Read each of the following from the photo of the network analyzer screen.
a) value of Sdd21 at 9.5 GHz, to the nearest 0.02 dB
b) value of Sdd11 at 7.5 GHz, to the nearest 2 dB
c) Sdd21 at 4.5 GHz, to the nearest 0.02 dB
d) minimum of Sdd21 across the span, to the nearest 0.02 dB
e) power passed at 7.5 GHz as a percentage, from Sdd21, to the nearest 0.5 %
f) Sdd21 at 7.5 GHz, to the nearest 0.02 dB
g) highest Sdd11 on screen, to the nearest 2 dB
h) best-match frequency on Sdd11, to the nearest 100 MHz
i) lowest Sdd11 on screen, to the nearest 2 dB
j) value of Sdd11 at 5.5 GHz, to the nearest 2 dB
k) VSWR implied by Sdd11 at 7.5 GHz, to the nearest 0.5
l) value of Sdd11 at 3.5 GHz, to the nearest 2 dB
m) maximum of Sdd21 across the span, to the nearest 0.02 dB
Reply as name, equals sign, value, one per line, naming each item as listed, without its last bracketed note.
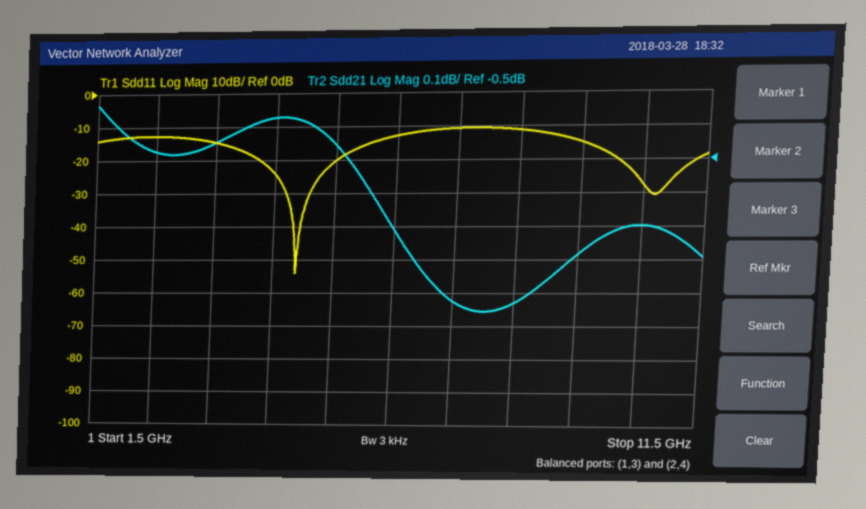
value of Sdd21 at 9.5 GHz, to the nearest 0.02 dB = -0.78 dB
value of Sdd11 at 7.5 GHz, to the nearest 2 dB = -10 dB
Sdd21 at 4.5 GHz, to the nearest 0.02 dB = -0.38 dB
minimum of Sdd21 across the span, to the nearest 0.02 dB = -0.96 dB
power passed at 7.5 GHz as a percentage, from Sdd21, to the nearest 0.5 % = 81.0 %
Sdd21 at 7.5 GHz, to the nearest 0.02 dB = -0.92 dB
highest Sdd11 on screen, to the nearest 2 dB = -10 dB
best-match frequency on Sdd11, to the nearest 100 MHz = 4.9 GHz
lowest Sdd11 on screen, to the nearest 2 dB = -54 dB
value of Sdd11 at 5.5 GHz, to the nearest 2 dB = -20 dB
VSWR implied by Sdd11 at 7.5 GHz, to the nearest 0.5 = 2.0
value of Sdd11 at 3.5 GHz, to the nearest 2 dB = -14 dB
maximum of Sdd21 across the span, to the nearest 0.02 dB = -0.34 dB
